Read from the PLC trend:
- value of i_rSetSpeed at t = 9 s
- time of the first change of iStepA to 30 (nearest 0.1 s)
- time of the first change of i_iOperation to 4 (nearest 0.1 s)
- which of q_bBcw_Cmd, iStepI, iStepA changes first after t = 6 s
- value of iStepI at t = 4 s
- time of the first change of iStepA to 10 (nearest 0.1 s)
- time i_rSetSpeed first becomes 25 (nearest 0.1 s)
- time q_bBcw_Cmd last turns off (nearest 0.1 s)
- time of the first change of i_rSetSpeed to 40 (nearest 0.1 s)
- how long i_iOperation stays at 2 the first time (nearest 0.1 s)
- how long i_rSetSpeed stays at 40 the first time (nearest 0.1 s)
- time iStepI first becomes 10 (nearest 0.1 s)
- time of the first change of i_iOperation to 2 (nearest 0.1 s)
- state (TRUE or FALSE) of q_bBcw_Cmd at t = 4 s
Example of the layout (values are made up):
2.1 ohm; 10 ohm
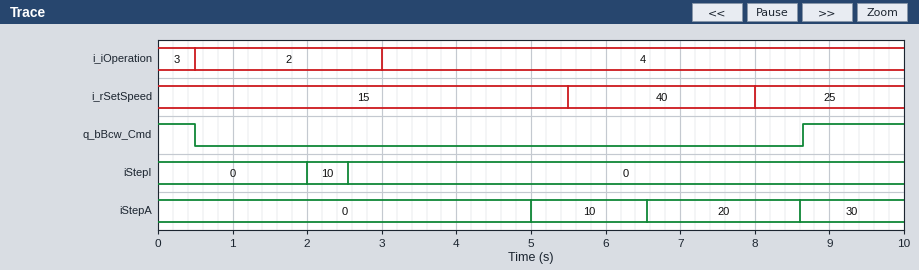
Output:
25; 8.6 s; 3.0 s; iStepA; 0; 5.0 s; 8.0 s; 0.5 s; 5.5 s; 2.5 s; 2.5 s; 2.0 s; 0.5 s; FALSE
